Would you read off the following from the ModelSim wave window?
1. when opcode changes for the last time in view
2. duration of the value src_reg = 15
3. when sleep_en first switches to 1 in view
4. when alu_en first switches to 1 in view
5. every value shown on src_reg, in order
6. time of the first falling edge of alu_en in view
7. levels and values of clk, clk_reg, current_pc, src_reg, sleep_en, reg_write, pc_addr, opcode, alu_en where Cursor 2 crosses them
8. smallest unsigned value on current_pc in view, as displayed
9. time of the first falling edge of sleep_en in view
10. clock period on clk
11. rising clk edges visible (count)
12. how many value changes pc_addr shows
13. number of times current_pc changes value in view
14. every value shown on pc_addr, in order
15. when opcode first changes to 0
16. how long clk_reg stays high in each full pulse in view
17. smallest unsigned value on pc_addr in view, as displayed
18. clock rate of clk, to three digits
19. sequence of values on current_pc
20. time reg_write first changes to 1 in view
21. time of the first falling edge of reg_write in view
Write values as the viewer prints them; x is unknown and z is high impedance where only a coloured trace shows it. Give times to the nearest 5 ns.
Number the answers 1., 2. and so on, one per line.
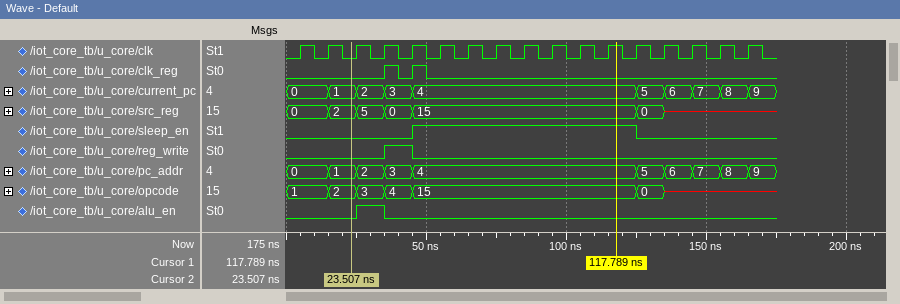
1. 135 ns
2. 80 ns
3. 45 ns
4. 25 ns
5. 0, 2, 5, 0, 15, 0, x
6. 35 ns
7. clk=0, clk_reg=0, current_pc=1, src_reg=2, sleep_en=0, reg_write=0, pc_addr=1, opcode=2, alu_en=0
8. 0
9. 125 ns
10. 10 ns
11. 17
12. 9
13. 9
14. 0, 1, 2, 3, 4, 5, 6, 7, 8, 9
15. 125 ns
16. 5 ns, 5 ns
17. 0
18. 100 MHz
19. 0, 1, 2, 3, 4, 5, 6, 7, 8, 9
20. 35 ns
21. 45 ns
